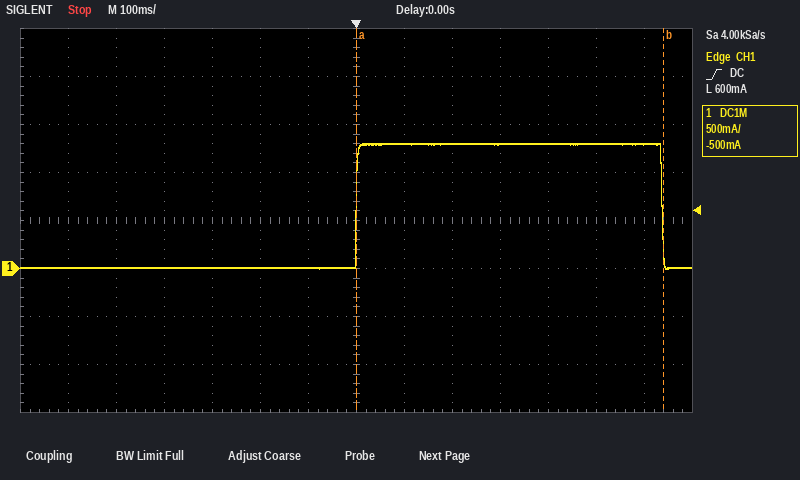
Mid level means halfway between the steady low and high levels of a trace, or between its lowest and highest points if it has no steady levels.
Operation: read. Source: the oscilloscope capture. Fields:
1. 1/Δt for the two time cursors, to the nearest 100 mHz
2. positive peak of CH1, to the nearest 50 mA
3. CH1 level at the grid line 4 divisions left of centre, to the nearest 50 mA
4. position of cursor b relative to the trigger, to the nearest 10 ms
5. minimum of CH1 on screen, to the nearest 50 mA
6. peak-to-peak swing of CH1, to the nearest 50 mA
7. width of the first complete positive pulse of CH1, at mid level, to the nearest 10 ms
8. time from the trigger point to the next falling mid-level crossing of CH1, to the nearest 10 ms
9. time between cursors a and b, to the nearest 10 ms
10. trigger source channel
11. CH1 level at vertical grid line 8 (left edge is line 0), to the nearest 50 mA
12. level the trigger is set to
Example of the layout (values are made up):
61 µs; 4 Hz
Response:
1.6 Hz; 1.30 A; 0 mA; +640 ms; 0 mA; 1.30 A; 640 ms; 640 ms; 640 ms; CH1; 1.30 A; 600 mA
